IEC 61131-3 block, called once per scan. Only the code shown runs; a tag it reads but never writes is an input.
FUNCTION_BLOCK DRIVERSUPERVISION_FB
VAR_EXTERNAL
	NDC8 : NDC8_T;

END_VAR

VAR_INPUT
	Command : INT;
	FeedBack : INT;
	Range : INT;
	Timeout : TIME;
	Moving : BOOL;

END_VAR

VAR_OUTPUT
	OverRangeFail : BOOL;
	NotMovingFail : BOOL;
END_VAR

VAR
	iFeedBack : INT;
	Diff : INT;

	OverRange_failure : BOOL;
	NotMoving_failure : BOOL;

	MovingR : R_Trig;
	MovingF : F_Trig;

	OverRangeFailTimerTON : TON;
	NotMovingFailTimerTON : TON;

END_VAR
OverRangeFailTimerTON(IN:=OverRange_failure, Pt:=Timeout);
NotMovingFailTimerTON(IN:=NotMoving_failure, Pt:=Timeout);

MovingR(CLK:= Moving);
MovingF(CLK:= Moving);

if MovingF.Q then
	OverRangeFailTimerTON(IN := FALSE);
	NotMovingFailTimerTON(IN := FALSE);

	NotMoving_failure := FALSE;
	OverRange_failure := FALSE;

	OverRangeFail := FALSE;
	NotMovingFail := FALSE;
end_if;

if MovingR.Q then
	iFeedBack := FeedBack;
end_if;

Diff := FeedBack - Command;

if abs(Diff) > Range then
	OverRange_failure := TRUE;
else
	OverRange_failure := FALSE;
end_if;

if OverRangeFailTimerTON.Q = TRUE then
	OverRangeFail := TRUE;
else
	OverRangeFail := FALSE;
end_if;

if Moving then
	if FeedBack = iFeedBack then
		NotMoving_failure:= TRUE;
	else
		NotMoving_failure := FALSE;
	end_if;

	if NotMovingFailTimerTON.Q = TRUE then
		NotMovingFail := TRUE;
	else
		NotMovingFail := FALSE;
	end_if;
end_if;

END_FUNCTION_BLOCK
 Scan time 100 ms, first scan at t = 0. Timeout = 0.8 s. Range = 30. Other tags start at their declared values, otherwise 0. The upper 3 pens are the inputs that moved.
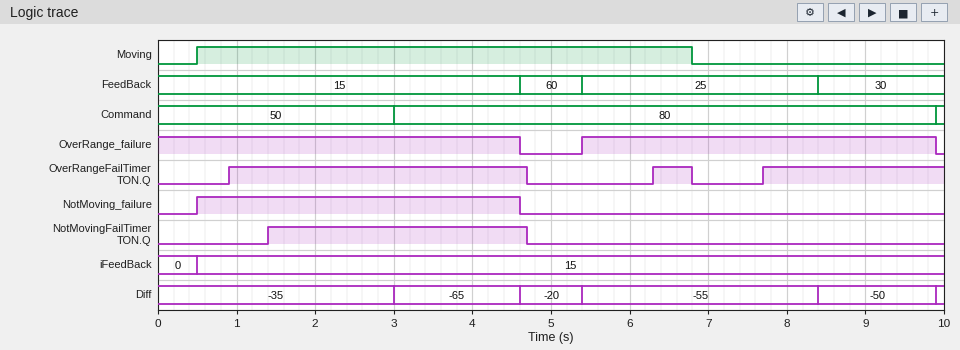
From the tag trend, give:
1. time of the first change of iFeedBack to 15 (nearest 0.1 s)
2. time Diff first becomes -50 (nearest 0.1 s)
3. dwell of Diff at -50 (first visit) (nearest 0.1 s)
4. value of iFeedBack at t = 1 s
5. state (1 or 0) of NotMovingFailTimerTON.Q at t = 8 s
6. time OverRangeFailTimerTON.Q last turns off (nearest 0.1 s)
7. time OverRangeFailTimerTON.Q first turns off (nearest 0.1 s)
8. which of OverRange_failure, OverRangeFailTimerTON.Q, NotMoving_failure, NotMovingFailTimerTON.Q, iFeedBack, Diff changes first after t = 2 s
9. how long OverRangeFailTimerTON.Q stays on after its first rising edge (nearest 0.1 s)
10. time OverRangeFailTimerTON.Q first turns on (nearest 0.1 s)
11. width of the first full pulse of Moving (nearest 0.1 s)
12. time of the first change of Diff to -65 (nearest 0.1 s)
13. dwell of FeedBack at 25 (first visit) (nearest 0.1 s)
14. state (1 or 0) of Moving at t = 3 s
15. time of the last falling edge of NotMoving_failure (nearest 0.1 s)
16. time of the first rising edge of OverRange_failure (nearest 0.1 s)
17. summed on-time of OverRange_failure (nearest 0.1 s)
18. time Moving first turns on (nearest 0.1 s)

0.5 s
8.4 s
1.5 s
15
0
6.8 s
4.7 s
Diff
3.8 s
0.9 s
6.3 s
3.0 s
3.0 s
1
4.6 s
5.4 s
9.1 s
0.5 s
